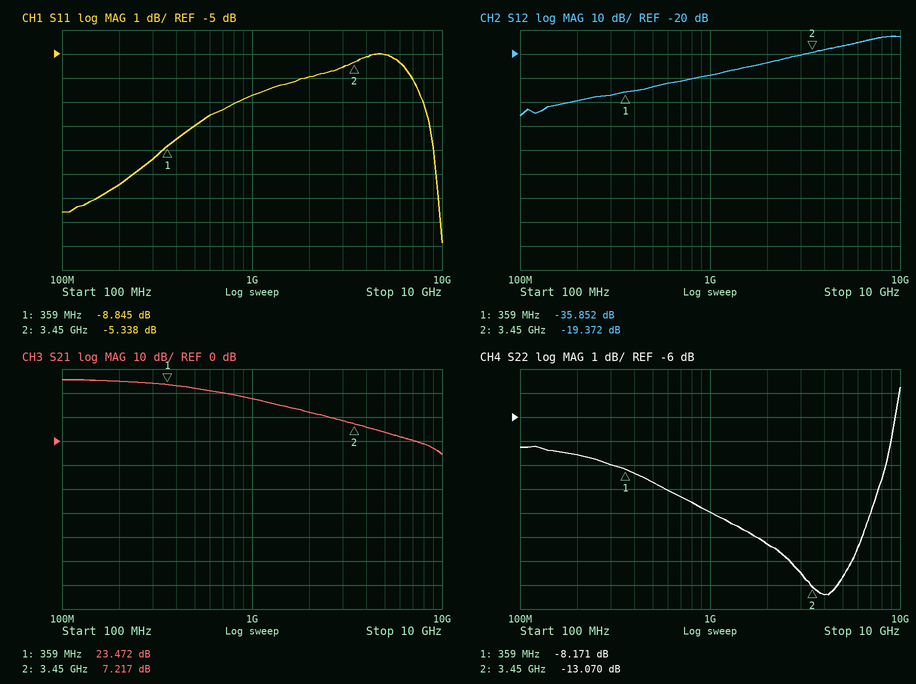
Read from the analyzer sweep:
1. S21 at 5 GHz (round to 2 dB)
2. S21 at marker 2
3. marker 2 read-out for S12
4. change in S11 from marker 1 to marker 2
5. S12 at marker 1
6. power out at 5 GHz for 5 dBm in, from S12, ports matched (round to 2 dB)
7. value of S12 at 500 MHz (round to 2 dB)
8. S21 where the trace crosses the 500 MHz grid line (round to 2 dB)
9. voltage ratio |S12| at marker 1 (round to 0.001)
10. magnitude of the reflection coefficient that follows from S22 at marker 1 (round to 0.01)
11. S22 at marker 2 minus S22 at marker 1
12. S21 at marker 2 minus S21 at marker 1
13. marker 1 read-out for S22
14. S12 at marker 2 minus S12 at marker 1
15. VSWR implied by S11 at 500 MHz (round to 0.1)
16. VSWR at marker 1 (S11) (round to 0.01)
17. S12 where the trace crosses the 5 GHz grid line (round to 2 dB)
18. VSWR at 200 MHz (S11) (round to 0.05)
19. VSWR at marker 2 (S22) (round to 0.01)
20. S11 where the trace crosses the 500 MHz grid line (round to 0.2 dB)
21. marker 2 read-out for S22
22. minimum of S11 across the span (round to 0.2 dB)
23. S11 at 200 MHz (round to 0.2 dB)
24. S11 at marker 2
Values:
4 dB
7.217 dB
-19.372 dB
3.507 dB
-35.852 dB
-12 dBm
-34 dB
22 dB
0.016
0.39
-4.899 dB
-16.255 dB
-8.171 dB
16.480 dB
2.3
2.13
-16 dB
1.85
1.57
-8.0 dB
-13.070 dB
-12.8 dB
-10.4 dB
-5.338 dB
